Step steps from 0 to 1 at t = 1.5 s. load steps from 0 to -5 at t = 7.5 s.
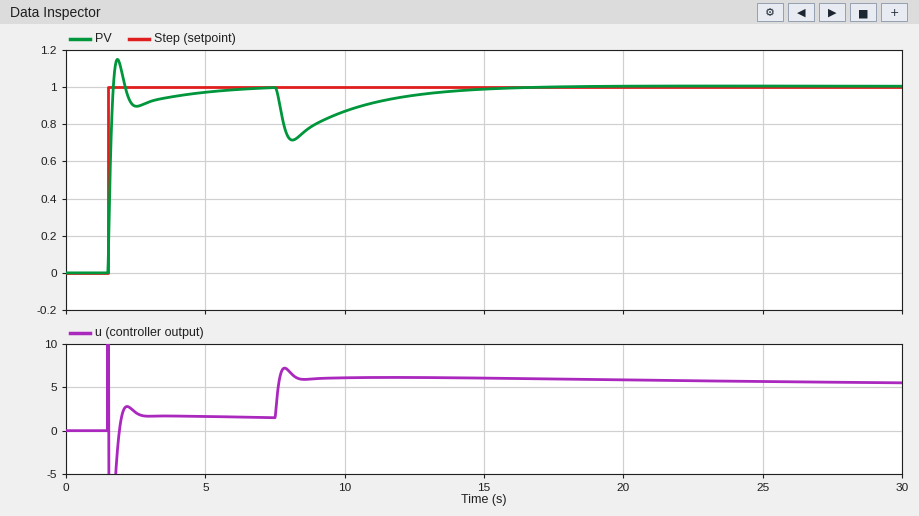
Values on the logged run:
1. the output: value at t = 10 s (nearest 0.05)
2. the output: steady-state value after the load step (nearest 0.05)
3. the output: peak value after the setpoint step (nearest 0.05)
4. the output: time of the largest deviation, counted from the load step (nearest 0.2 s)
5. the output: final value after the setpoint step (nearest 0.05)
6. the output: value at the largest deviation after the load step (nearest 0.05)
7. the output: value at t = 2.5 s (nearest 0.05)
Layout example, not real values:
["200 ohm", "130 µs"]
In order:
["0.85", "1.00", "1.15", "0.6 s", "1.00", "0.70", "0.90"]
